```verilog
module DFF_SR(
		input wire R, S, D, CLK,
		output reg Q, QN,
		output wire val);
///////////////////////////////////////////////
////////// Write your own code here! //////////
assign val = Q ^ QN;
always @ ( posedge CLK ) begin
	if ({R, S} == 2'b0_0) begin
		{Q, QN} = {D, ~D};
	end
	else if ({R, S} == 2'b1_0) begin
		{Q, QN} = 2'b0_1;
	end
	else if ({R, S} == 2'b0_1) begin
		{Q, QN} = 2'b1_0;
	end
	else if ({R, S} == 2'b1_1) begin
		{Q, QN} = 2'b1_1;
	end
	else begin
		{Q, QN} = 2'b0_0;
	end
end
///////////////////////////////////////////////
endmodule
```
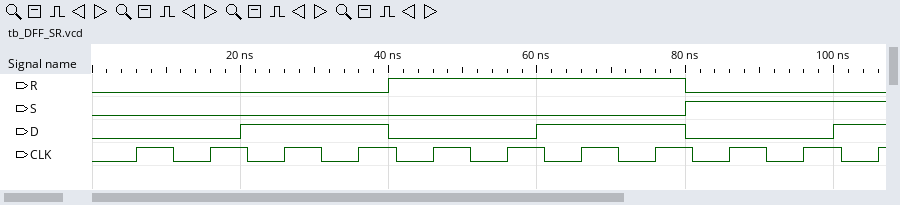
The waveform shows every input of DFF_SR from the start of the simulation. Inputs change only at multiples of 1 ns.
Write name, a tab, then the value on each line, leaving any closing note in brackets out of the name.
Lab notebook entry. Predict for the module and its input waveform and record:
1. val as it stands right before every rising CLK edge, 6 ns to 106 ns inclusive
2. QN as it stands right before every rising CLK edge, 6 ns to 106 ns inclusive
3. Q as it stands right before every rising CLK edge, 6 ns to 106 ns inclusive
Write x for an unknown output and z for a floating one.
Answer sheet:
val as it stands right before every rising CLK edge, 6 ns to 106 ns inclusive	x 1 1 1 1 1 1 1 1 1 1
QN as it stands right before every rising CLK edge, 6 ns to 106 ns inclusive	x 1 1 0 0 1 1 1 1 0 0
Q as it stands right before every rising CLK edge, 6 ns to 106 ns inclusive	x 0 0 1 1 0 0 0 0 1 1
